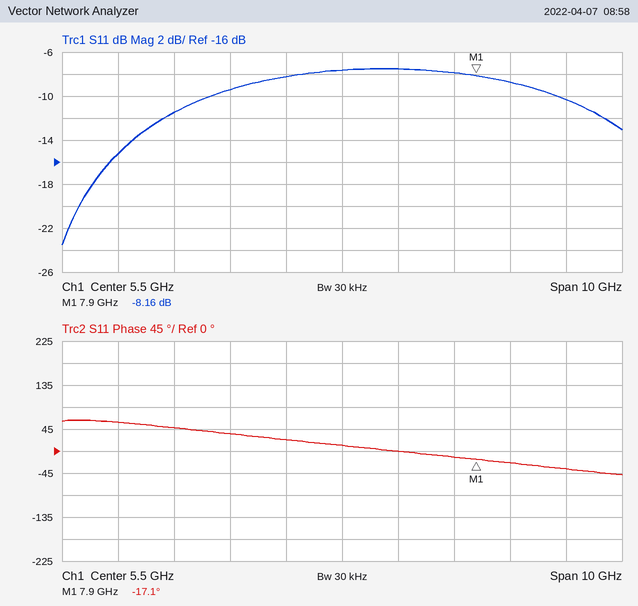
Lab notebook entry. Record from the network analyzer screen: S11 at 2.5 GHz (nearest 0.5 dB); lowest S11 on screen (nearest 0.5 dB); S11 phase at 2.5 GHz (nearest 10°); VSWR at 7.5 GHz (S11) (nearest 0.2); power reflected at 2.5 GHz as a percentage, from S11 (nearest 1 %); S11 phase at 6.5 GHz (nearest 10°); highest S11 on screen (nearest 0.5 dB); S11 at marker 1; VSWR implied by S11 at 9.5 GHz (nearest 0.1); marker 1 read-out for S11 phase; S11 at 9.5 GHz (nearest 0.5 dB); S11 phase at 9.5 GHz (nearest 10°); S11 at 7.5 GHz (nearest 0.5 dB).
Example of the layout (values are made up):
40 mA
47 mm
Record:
-11.5 dB
-23.5 dB
50°
2.4
7 %
0°
-7.5 dB
-8.16 dB
1.9
-17.1°
-10.5 dB
-40°
-8.0 dB
